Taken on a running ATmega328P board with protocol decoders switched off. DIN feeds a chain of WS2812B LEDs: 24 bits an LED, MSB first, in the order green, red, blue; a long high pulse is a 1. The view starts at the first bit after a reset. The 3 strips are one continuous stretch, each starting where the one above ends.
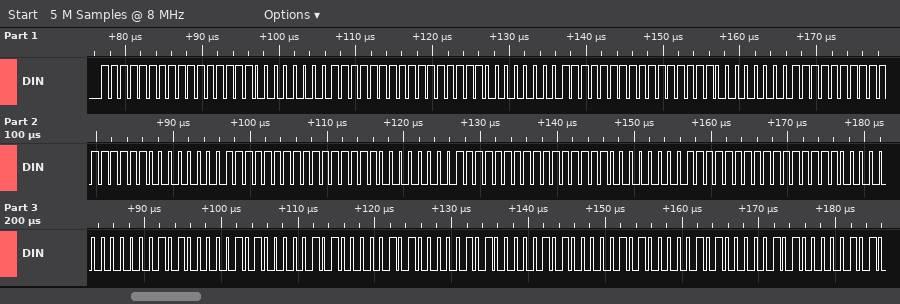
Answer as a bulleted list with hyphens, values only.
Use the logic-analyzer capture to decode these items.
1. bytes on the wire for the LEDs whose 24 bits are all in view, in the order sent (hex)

- FF FF 00 FF FF 00 FF FF 00 FF FF 00 FF FF 00 FF FF 00 FF FF 00 0A 0A 0A 0A 0A 0A 0A 0A 0A
